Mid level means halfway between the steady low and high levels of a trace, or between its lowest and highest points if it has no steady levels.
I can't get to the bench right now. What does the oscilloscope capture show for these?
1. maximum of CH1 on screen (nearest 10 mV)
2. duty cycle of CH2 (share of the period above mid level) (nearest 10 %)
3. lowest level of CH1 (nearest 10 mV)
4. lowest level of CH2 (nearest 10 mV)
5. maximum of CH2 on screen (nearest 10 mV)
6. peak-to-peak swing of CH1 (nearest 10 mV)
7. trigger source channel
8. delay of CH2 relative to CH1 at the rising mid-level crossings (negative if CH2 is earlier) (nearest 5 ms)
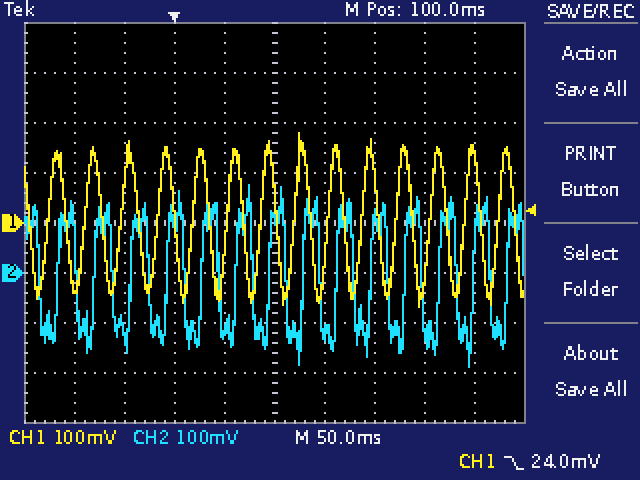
180 mV
50 %
-170 mV
-190 mV
180 mV
350 mV
CH1
+10 ms
